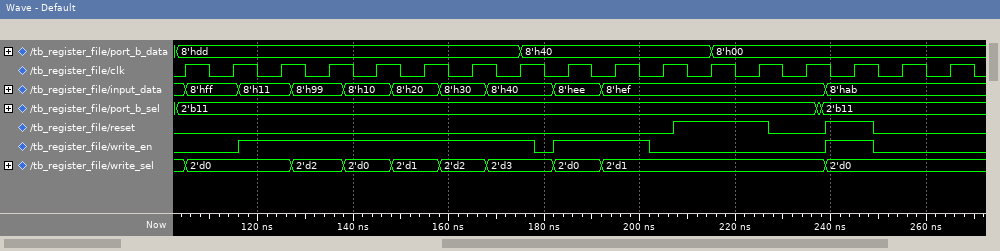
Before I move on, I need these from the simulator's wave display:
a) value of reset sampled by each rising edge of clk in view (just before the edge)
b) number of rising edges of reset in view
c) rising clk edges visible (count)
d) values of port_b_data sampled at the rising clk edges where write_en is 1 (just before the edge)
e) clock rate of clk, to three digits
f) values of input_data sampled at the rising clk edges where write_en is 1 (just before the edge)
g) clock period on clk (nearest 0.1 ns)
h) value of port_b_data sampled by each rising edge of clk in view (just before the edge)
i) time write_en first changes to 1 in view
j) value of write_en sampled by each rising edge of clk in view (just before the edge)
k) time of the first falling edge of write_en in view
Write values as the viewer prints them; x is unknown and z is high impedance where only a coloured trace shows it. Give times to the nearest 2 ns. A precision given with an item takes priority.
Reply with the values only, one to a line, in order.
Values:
0 0 0 0 0 0 0 0 0 0 0 1 1 0 1 0 0
2
17
8'hdd, 8'hdd, 8'hdd, 8'hdd, 8'hdd, 8'hdd, 8'h40, 8'h40, 8'h00
100 MHz
8'h11, 8'h99, 8'h10, 8'h20, 8'h30, 8'h40, 8'hee, 8'hef, 8'hab
10 ns
8'hdd, 8'hdd, 8'hdd, 8'hdd, 8'hdd, 8'hdd, 8'hdd, 8'hdd, 8'h40, 8'h40, 8'h40, 8'h40, 8'h00, 8'h00, 8'h00, 8'h00, 8'h00
116 ns
0 0 1 1 1 1 1 1 1 1 0 0 0 0 1 0 0
178 ns
